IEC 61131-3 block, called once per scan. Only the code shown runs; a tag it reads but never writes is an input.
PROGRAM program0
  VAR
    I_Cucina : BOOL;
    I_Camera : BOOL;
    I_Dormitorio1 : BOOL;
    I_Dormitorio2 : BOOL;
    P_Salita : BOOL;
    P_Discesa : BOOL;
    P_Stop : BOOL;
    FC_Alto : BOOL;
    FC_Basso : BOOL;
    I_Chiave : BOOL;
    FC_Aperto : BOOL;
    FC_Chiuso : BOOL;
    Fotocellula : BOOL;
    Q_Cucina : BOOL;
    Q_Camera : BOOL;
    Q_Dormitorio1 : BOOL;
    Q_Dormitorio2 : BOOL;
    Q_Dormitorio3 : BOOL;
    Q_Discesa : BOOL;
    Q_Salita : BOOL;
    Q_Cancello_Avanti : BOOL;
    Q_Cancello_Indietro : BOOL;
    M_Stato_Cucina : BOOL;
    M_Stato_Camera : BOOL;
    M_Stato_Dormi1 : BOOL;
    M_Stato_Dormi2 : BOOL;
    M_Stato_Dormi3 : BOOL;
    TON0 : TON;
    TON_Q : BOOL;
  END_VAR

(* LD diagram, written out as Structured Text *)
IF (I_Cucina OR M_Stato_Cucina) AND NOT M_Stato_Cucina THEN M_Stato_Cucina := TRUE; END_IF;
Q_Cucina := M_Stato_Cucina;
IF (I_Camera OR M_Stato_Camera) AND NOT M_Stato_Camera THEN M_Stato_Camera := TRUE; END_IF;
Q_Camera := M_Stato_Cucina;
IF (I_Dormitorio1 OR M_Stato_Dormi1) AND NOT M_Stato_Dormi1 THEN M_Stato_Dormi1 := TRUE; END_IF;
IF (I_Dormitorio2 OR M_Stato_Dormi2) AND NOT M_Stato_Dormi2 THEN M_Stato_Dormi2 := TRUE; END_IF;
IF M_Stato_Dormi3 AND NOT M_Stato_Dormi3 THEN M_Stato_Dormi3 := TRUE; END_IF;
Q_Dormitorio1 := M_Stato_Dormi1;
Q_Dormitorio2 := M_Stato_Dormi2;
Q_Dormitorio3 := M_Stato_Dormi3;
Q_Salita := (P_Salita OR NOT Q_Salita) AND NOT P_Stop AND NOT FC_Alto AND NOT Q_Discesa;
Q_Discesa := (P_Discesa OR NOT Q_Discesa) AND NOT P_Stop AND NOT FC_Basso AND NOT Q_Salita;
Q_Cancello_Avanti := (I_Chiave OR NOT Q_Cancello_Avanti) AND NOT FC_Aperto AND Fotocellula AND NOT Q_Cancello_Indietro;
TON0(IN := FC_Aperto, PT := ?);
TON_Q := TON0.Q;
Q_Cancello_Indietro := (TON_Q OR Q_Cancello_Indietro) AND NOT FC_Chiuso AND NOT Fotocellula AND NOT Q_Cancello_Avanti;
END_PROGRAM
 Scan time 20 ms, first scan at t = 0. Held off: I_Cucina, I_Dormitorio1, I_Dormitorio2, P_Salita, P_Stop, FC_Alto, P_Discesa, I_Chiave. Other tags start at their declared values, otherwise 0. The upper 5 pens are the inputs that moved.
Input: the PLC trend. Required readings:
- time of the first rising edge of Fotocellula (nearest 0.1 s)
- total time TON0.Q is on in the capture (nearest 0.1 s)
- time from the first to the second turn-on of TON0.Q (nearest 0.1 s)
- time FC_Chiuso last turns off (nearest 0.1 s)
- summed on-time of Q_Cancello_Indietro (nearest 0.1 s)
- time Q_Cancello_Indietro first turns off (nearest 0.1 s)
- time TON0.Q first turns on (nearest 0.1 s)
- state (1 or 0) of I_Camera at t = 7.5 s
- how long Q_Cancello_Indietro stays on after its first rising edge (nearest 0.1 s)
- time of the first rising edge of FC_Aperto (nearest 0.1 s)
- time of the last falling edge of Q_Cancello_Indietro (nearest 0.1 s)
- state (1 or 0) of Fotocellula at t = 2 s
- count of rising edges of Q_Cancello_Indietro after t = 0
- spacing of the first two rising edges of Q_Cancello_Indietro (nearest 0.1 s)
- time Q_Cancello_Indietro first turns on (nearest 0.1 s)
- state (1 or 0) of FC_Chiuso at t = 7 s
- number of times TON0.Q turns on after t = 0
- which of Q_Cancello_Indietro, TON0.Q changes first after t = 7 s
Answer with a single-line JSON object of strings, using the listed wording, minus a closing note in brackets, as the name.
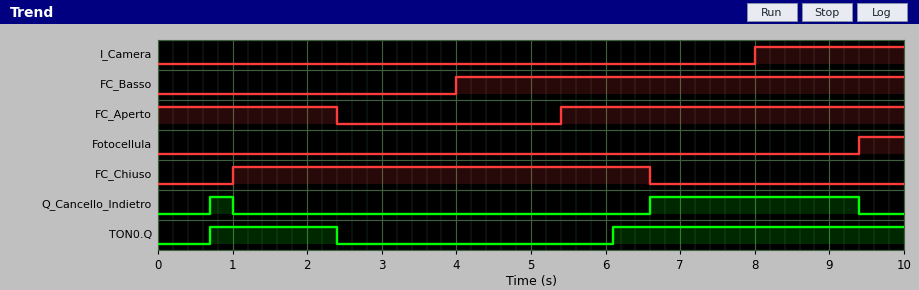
{"time of the first rising edge of Fotocellula": "9.4 s", "total time TON0.Q is on in the capture": "5.6 s", "time from the first to the second turn-on of TON0.Q": "5.4 s", "time FC_Chiuso last turns off": "6.6 s", "summed on-time of Q_Cancello_Indietro": "3.1 s", "time Q_Cancello_Indietro first turns off": "1.0 s", "time TON0.Q first turns on": "0.7 s", "state (1 or 0) of I_Camera at t = 7.5 s": "0", "how long Q_Cancello_Indietro stays on after its first rising edge": "0.3 s", "time of the first rising edge of FC_Aperto": "5.4 s", "time of the last falling edge of Q_Cancello_Indietro": "9.4 s", "state (1 or 0) of Fotocellula at t = 2 s": "0", "count of rising edges of Q_Cancello_Indietro after t = 0": "2", "spacing of the first two rising edges of Q_Cancello_Indietro": "5.9 s", "time Q_Cancello_Indietro first turns on": "0.7 s", "state (1 or 0) of FC_Chiuso at t = 7 s": "0", "number of times TON0.Q turns on after t = 0": "2", "which of Q_Cancello_Indietro, TON0.Q changes first after t = 7 s": "Q_Cancello_Indietro"}
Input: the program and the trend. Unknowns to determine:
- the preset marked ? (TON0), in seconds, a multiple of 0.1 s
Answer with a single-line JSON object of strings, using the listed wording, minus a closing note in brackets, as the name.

{"the preset marked ? (TON0), in seconds, a multiple of 0.1 s": "0.7 s"}
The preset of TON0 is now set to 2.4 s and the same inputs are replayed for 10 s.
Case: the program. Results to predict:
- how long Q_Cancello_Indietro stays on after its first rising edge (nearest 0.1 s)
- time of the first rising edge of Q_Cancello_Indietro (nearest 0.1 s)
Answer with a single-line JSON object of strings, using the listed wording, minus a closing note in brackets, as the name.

{"how long Q_Cancello_Indietro stays on after its first rising edge": "1.6 s", "time of the first rising edge of Q_Cancello_Indietro": "7.8 s"}
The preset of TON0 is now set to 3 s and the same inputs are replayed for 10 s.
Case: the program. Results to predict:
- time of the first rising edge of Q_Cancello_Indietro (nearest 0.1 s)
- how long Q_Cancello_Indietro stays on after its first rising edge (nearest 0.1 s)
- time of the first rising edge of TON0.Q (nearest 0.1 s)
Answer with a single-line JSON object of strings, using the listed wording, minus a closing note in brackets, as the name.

{"time of the first rising edge of Q_Cancello_Indietro": "8.4 s", "how long Q_Cancello_Indietro stays on after its first rising edge": "1.0 s", "time of the first rising edge of TON0.Q": "8.4 s"}
